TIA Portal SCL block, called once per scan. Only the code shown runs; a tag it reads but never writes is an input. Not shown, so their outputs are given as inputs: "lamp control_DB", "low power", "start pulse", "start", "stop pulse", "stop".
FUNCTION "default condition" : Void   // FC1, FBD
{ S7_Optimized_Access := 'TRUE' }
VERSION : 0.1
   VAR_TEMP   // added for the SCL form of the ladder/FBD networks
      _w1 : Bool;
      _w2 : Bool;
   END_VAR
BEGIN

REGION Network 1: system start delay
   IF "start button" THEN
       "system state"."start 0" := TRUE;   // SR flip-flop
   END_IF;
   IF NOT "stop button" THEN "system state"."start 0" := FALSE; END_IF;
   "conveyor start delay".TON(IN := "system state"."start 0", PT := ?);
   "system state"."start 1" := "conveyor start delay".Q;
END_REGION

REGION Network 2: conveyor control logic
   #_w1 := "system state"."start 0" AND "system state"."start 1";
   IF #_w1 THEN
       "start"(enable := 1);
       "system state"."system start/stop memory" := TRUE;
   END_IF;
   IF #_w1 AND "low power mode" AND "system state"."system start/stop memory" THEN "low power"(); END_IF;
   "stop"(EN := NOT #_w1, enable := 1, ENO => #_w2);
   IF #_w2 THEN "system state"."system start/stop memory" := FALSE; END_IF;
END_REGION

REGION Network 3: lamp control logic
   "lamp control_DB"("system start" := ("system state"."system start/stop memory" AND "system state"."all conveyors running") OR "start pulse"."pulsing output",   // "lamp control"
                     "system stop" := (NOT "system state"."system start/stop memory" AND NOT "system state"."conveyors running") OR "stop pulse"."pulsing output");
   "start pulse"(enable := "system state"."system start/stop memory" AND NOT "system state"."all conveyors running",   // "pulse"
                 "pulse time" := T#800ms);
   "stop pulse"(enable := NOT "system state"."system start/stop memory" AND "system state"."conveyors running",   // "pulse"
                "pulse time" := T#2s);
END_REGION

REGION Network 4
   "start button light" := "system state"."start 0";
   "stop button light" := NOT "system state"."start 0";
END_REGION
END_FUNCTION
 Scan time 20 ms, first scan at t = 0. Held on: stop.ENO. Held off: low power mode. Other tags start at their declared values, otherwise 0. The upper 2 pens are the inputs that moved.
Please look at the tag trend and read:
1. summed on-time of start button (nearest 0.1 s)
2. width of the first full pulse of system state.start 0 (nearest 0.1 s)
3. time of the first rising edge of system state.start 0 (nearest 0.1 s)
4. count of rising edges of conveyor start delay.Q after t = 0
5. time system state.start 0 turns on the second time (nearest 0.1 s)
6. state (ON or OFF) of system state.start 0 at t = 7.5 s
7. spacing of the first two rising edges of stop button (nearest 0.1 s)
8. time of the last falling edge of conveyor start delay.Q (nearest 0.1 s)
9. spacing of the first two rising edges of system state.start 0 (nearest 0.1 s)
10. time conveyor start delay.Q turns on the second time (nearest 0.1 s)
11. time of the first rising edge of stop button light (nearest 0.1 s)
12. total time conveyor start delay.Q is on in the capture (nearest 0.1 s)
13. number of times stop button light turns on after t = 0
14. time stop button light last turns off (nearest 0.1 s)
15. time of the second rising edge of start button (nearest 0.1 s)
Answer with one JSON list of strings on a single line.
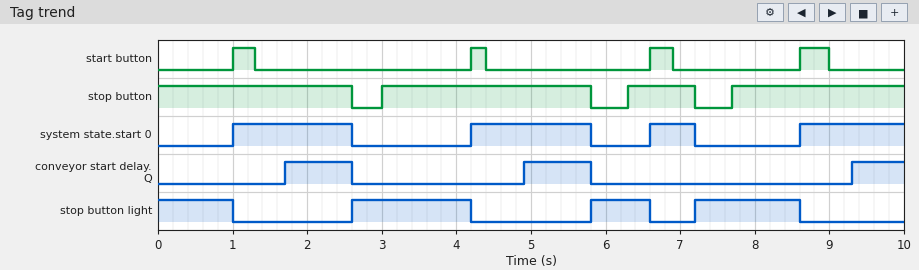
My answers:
["1.2 s", "1.6 s", "1.0 s", "3", "4.2 s", "OFF", "3.3 s", "5.8 s", "3.2 s", "4.9 s", "2.6 s", "2.5 s", "3", "8.6 s", "4.2 s"]
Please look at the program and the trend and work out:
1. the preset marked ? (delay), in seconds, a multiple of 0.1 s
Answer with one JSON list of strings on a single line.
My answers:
["0.7 s"]
